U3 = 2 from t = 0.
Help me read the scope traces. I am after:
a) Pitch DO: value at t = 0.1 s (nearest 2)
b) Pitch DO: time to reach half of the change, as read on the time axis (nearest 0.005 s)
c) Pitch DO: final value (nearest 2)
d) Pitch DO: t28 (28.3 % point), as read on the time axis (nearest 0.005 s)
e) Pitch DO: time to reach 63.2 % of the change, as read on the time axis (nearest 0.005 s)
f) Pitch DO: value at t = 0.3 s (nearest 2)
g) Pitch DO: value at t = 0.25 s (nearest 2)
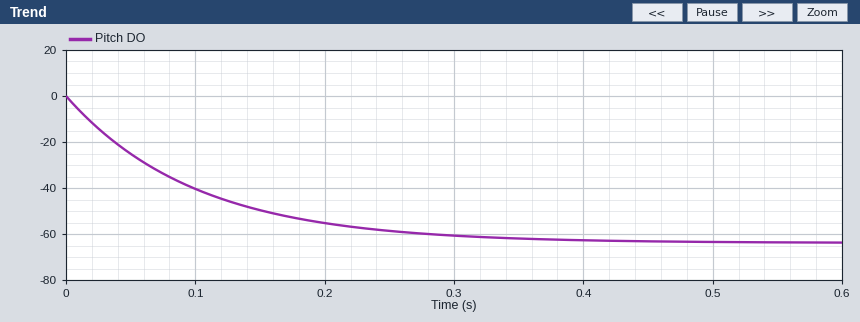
-40
0.070 s
-64
0.035 s
0.100 s
-60
-58
